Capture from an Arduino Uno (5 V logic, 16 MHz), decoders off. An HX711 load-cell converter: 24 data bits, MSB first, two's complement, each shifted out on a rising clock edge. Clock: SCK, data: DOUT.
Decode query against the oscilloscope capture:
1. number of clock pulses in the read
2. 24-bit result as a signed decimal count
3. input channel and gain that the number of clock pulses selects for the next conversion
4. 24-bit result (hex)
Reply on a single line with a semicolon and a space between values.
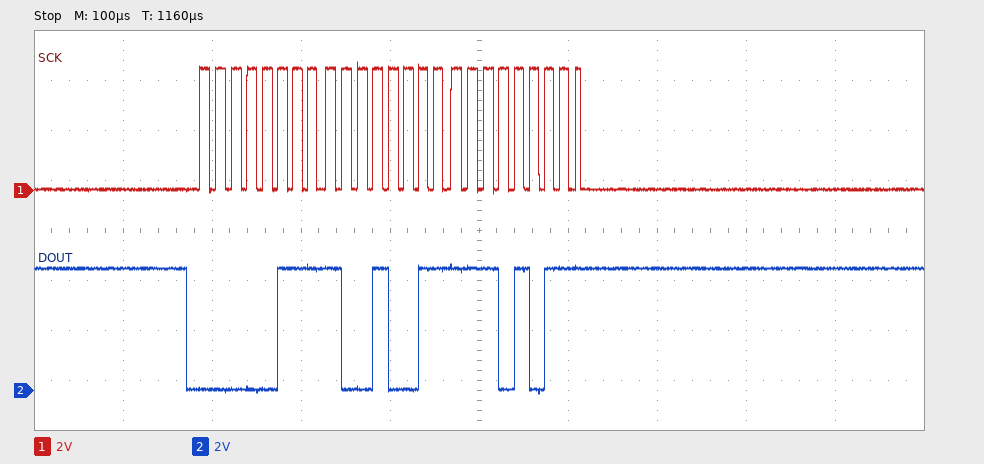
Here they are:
25; 496619; channel A, gain 128; 0x0793EB
